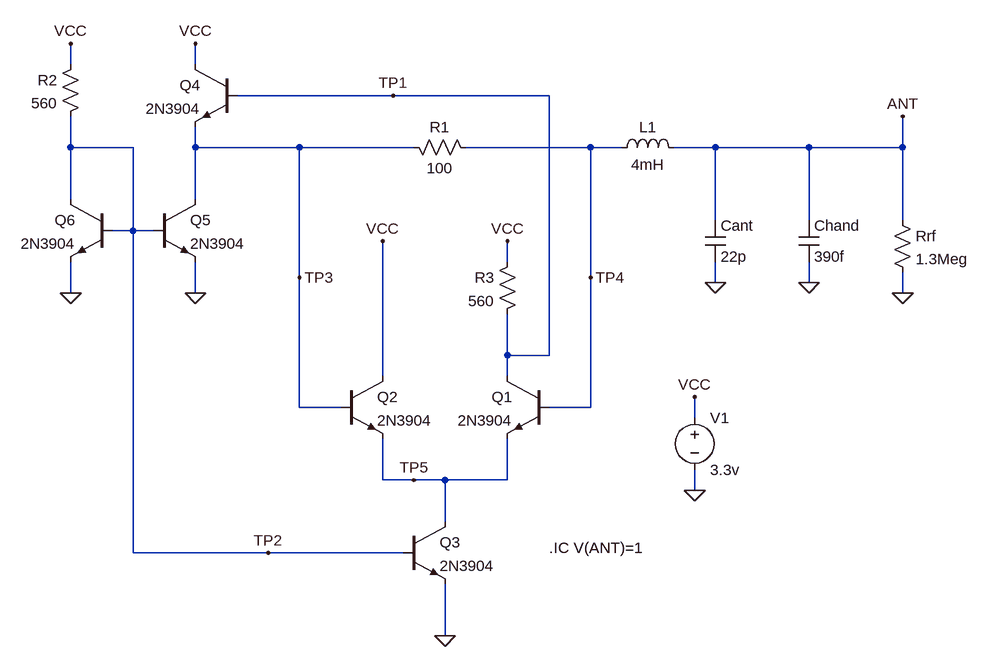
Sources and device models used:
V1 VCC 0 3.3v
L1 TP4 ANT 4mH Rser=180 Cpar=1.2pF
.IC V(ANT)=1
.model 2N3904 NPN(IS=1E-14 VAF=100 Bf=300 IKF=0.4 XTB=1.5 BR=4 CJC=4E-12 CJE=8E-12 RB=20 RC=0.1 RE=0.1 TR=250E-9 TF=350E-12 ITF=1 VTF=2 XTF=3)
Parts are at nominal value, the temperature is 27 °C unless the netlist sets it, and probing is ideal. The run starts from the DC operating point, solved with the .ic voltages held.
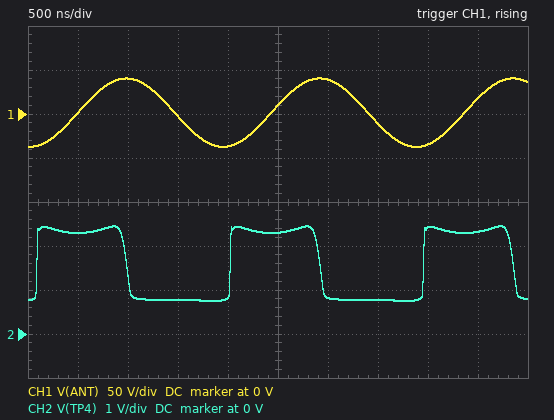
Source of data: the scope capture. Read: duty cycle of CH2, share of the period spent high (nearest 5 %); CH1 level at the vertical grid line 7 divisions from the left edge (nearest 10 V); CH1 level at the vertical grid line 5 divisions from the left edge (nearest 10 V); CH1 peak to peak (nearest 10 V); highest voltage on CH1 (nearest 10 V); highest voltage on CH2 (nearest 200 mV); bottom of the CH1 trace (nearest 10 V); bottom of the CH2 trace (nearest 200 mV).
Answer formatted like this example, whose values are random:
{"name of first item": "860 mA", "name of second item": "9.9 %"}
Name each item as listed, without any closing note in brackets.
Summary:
{"duty cycle of CH2, share of the period spent high": "45 %", "CH1 level at the vertical grid line 7 divisions from the left edge": "-10 V", "CH1 level at the vertical grid line 5 divisions from the left edge": "10 V", "CH1 peak to peak": "80 V", "highest voltage on CH1": "40 V", "highest voltage on CH2": "2.4 V", "bottom of the CH1 trace": "-40 V", "bottom of the CH2 trace": "800 mV"}
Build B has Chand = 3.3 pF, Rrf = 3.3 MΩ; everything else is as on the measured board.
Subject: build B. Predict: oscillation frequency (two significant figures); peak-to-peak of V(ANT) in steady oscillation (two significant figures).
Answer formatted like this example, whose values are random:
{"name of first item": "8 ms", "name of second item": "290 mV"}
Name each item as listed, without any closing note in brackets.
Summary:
{"oscillation frequency": "490 kHz", "peak-to-peak of V(ANT) in steady oscillation": "96 V"}
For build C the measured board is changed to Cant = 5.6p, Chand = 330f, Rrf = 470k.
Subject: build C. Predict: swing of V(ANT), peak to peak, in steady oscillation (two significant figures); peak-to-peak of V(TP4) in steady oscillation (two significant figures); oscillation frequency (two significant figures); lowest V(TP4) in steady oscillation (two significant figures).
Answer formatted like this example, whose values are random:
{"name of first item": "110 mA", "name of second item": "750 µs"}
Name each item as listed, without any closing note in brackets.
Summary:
{"swing of V(ANT), peak to peak, in steady oscillation": "17 V", "peak-to-peak of V(TP4) in steady oscillation": "1.1 V", "oscillation frequency": "940 kHz", "lowest V(TP4) in steady oscillation": "820 mV"}
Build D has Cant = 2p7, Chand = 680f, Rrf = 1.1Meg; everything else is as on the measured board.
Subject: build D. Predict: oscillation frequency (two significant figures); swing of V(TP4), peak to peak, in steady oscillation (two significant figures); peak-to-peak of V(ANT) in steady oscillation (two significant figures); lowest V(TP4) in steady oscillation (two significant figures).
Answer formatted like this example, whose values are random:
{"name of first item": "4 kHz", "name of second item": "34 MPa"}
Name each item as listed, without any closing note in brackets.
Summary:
{"oscillation frequency": "1.2 MHz", "swing of V(TP4), peak to peak, in steady oscillation": "1.3 V", "peak-to-peak of V(ANT) in steady oscillation": "31 V", "lowest V(TP4) in steady oscillation": "800 mV"}
